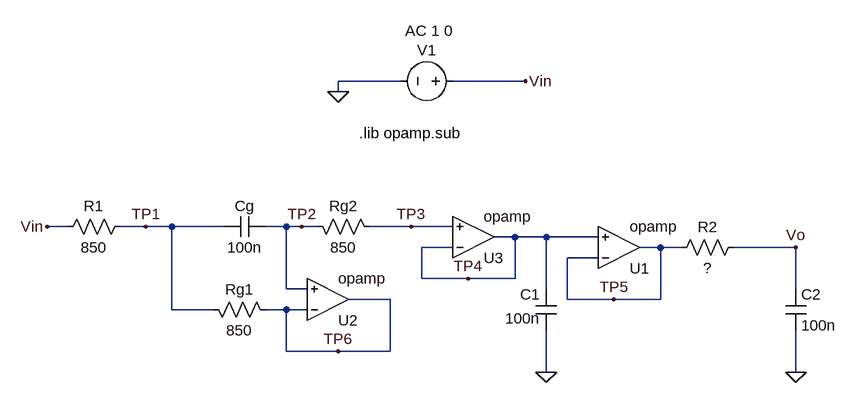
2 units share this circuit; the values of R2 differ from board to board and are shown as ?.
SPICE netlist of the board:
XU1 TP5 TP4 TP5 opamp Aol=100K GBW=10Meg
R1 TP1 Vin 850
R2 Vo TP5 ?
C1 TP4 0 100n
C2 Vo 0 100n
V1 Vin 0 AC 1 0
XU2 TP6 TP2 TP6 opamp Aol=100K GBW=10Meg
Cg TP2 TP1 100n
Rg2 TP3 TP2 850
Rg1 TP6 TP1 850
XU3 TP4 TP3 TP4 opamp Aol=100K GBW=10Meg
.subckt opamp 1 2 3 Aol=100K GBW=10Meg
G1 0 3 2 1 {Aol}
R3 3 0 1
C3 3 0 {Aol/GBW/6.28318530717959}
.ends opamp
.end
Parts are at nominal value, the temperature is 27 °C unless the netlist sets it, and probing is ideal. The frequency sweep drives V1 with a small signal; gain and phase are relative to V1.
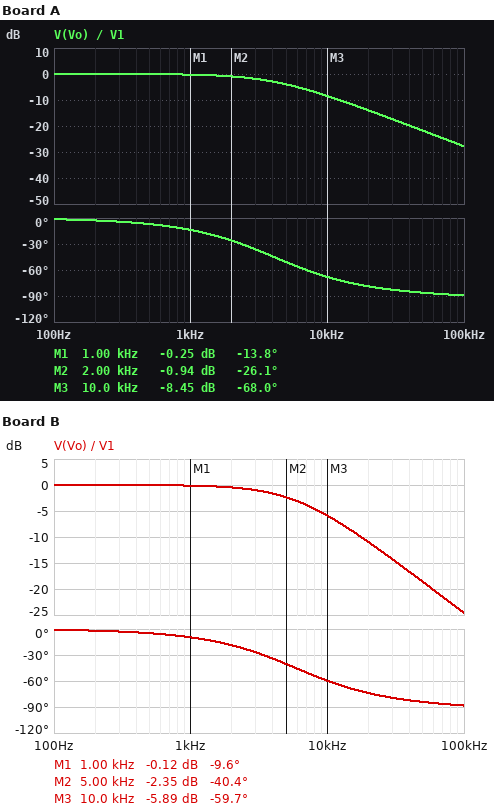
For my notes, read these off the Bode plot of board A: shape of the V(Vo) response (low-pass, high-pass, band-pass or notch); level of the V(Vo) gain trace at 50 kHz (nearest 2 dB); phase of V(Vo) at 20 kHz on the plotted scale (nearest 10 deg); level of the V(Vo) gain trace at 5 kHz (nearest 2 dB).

low-pass
-22 dB
-80 deg
-4 dB
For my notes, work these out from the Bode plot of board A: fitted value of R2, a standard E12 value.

390 Ω
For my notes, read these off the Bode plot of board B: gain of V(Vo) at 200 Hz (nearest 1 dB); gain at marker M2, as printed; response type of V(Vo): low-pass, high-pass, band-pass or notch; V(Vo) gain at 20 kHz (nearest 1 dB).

0 dB
-2.35 dB
low-pass
-11 dB
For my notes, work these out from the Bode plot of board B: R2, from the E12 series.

270 Ω
